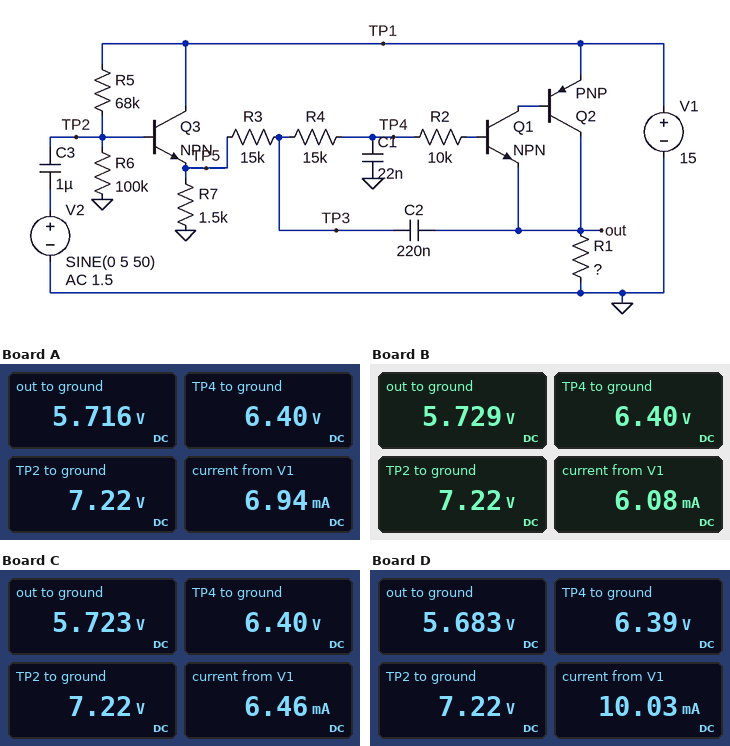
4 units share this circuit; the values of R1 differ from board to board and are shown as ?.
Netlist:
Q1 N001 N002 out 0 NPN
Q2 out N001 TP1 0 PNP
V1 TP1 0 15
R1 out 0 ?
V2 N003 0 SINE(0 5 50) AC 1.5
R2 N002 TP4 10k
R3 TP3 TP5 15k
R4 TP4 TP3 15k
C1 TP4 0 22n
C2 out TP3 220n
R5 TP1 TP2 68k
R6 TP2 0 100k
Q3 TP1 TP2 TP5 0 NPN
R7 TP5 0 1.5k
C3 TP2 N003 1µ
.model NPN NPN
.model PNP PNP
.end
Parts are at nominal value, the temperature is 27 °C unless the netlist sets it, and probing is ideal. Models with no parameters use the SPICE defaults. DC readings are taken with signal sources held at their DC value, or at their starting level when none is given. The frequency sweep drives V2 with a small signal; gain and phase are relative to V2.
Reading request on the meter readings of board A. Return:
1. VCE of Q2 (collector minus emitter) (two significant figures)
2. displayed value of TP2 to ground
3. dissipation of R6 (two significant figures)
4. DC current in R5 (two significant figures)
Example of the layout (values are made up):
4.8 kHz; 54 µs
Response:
-9.3 V; 7.22 V; 520 µW; 110 µA
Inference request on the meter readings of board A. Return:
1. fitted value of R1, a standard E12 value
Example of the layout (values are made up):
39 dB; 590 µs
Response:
2.2 kΩ
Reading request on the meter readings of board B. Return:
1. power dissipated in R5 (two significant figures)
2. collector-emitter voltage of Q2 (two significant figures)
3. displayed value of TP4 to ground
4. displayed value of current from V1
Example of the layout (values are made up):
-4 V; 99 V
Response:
890 µW; -9.3 V; 6.40 V; 6.08 mA
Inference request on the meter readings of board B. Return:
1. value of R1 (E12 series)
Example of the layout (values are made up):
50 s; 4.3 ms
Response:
3.3 kΩ
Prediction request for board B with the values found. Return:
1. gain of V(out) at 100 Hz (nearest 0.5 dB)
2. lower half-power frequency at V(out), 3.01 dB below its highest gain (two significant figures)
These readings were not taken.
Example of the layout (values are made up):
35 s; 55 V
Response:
3.0 dB; 63 Hz
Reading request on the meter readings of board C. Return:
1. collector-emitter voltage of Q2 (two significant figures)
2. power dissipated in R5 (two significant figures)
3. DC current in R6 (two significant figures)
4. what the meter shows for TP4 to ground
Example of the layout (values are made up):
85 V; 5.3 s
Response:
-9.3 V; 890 µW; 72 µA; 6.40 V
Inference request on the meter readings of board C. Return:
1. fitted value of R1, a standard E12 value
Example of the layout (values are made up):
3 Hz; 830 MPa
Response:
2.7 kΩ
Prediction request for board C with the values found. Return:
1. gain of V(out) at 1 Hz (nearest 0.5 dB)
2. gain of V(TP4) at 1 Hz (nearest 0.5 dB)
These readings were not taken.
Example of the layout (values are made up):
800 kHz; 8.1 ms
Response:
-14.0 dB; -14.0 dB
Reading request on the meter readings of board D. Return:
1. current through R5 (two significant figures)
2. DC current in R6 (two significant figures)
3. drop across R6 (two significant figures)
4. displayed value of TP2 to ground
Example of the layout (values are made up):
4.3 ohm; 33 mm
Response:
110 µA; 72 µA; 7.2 V; 7.22 V
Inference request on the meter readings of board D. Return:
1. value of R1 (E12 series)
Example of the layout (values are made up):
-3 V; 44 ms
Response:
1 kΩ
